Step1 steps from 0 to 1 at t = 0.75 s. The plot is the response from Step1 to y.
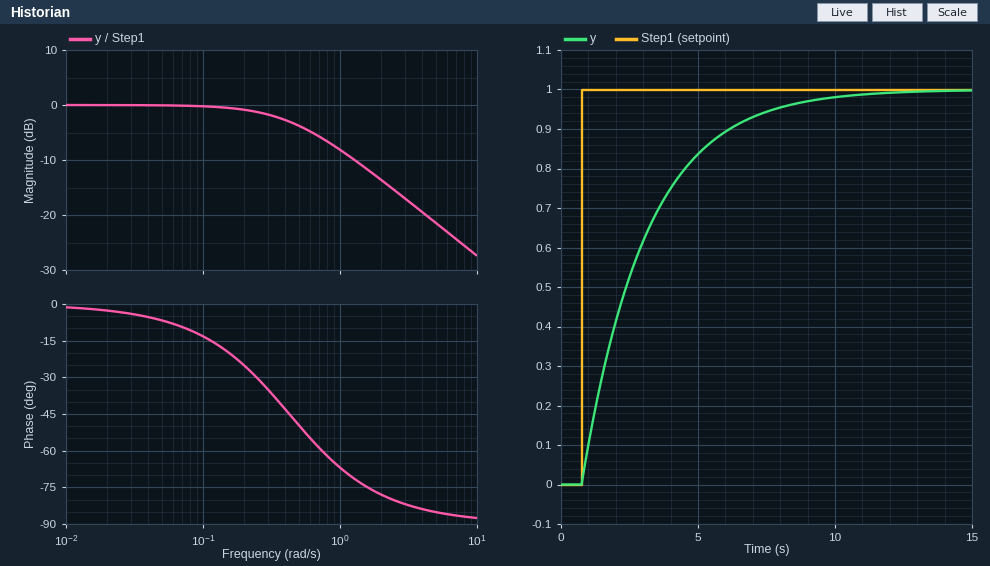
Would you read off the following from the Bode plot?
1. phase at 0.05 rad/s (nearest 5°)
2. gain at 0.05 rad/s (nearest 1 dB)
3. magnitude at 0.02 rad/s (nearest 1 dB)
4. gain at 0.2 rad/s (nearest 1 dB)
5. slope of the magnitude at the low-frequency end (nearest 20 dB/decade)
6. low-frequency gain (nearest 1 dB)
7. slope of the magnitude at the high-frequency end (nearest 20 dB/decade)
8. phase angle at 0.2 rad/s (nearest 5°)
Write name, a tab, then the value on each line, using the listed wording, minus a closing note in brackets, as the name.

phase at 0.05 rad/s	-5°
gain at 0.05 rad/s	0 dB
magnitude at 0.02 rad/s	0 dB
gain at 0.2 rad/s	-1 dB
slope of the magnitude at the low-frequency end	0 dB/decade
low-frequency gain	0 dB
slope of the magnitude at the high-frequency end	-20 dB/decade
phase angle at 0.2 rad/s	-25°
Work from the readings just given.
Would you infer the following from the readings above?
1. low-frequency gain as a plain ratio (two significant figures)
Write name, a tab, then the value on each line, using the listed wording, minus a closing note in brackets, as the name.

low-frequency gain as a plain ratio	1.0
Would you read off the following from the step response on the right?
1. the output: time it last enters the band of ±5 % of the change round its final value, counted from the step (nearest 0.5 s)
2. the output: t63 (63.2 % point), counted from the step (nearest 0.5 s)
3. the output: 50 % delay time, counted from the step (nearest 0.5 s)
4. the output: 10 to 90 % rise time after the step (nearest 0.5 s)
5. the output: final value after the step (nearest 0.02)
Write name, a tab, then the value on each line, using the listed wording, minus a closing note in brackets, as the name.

the output: time it last enters the band of ±5 % of the change round its final value, counted from the step	7.0 s
the output: t63 (63.2 % point), counted from the step	2.5 s
the output: 50 % delay time, counted from the step	1.5 s
the output: 10 to 90 % rise time after the step	5.0 s
the output: final value after the step	1.00
